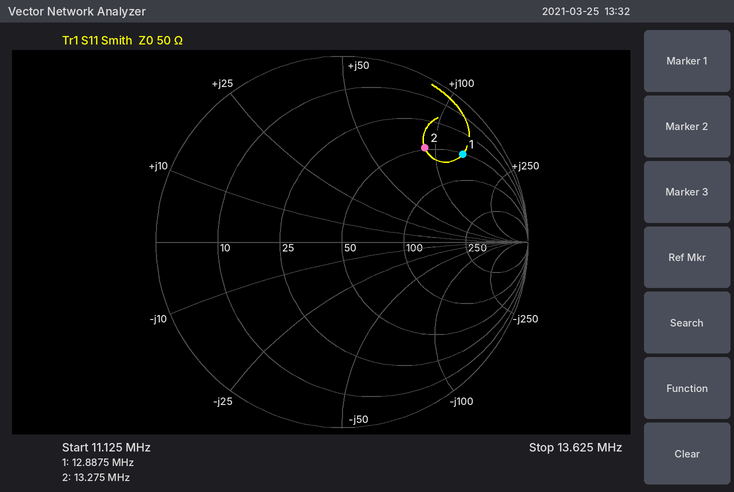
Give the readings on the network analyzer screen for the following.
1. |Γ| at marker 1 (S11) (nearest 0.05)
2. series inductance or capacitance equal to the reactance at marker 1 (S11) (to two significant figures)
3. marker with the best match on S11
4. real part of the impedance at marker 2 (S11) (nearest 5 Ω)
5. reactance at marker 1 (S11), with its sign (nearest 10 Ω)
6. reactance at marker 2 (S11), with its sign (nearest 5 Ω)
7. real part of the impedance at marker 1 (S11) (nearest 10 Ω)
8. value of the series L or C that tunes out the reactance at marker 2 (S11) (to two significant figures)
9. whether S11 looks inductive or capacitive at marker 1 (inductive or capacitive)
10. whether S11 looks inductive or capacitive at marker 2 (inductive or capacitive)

0.80
1.7 µH
marker 2
50 Ω
+140 Ω
+90 Ω
50 Ω
130 pF
inductive
inductive
